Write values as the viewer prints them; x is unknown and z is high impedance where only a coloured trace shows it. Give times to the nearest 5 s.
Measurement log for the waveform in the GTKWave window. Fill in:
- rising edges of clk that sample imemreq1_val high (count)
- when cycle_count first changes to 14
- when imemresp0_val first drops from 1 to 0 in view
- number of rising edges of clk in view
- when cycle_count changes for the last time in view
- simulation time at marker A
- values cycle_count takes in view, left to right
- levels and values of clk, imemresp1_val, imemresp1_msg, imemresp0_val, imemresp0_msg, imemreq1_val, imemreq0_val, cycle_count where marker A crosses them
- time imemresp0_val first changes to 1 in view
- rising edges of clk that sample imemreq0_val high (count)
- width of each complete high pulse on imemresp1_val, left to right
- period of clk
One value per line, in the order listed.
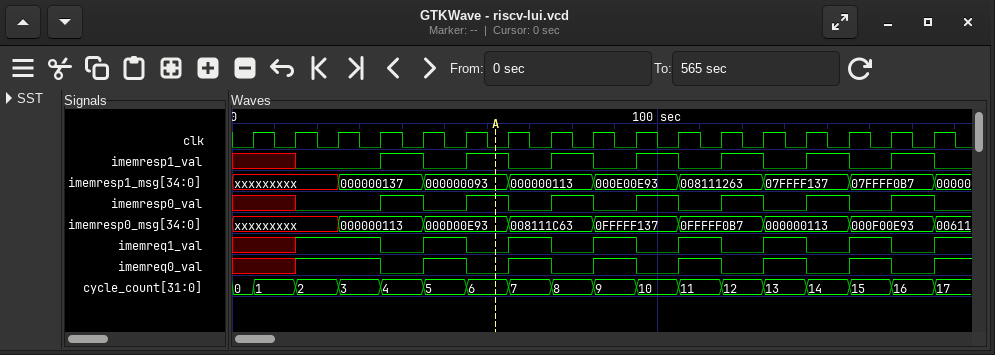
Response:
8
135 s
45 s
17
165 s
60 s
0, 1, 2, 3, 4, 5, 6, 7, 8, 9, 10, 11, 12, 13, 14, 15, 16, 17
clk=0, imemresp1_val=1, imemresp1_msg=000000093, imemresp0_val=1, imemresp0_msg=000D00E93, imemreq1_val=0, imemreq0_val=0, cycle_count=6
35 s
8
10 s, 10 s, 10 s, 10 s, 10 s, 10 s, 10 s
10 s
